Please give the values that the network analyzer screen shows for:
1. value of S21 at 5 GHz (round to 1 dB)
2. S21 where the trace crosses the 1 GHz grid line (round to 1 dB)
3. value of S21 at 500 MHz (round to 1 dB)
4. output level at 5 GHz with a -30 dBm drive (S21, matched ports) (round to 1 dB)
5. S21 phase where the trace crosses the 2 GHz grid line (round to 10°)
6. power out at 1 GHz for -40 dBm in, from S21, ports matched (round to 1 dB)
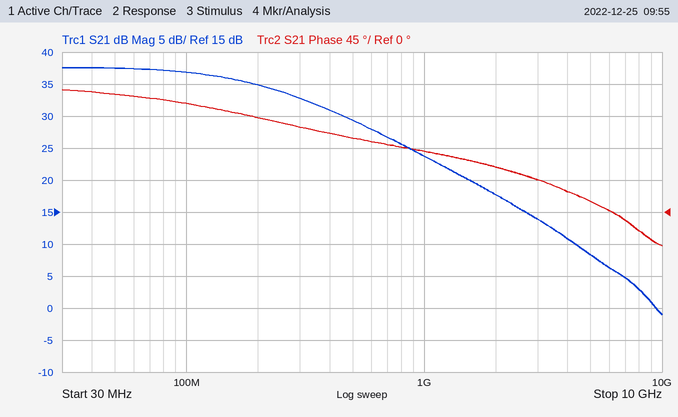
8 dB
24 dB
29 dB
-22 dBm
60°
-16 dBm
